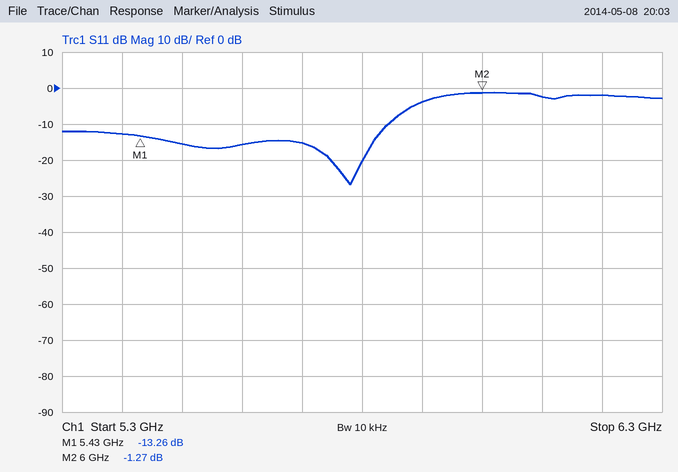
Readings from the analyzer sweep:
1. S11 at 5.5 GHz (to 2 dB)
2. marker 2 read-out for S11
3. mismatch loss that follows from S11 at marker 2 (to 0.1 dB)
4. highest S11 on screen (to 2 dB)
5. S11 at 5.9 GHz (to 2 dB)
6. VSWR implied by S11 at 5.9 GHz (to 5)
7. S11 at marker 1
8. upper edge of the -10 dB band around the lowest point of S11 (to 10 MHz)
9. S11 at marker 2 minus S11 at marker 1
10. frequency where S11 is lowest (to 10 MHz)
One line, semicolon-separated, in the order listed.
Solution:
-16 dB; -1.27 dB; 6.0 dB; -2 dB; -4 dB; 5; -13.26 dB; 5.84 GHz; 11.99 dB; 5.78 GHz
